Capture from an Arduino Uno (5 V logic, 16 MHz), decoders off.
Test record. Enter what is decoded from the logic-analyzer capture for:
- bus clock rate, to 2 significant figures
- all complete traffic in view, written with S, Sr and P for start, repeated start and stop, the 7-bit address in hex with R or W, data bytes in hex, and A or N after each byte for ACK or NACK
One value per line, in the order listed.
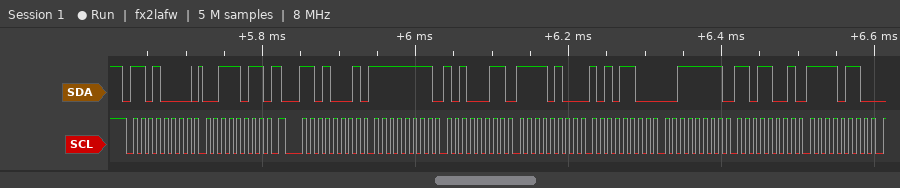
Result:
100 kHz
S 68W A 3B A Sr 68R A FF A A3 A F4 A AC A 3F A D9 A F6 A
